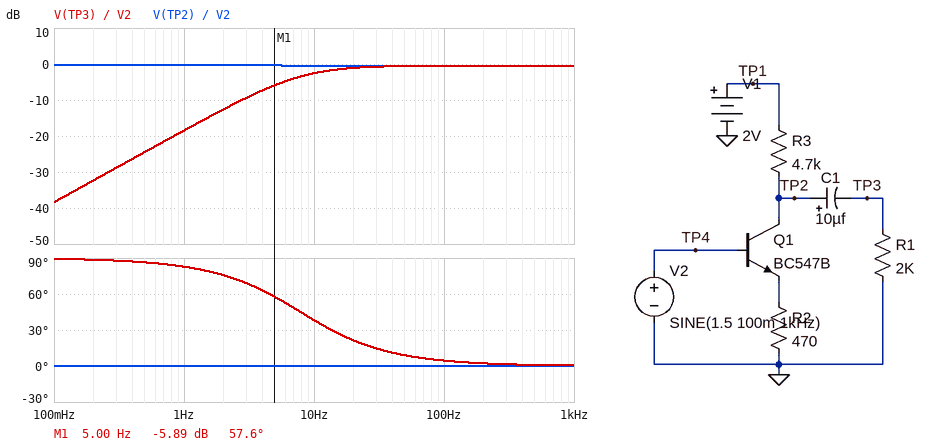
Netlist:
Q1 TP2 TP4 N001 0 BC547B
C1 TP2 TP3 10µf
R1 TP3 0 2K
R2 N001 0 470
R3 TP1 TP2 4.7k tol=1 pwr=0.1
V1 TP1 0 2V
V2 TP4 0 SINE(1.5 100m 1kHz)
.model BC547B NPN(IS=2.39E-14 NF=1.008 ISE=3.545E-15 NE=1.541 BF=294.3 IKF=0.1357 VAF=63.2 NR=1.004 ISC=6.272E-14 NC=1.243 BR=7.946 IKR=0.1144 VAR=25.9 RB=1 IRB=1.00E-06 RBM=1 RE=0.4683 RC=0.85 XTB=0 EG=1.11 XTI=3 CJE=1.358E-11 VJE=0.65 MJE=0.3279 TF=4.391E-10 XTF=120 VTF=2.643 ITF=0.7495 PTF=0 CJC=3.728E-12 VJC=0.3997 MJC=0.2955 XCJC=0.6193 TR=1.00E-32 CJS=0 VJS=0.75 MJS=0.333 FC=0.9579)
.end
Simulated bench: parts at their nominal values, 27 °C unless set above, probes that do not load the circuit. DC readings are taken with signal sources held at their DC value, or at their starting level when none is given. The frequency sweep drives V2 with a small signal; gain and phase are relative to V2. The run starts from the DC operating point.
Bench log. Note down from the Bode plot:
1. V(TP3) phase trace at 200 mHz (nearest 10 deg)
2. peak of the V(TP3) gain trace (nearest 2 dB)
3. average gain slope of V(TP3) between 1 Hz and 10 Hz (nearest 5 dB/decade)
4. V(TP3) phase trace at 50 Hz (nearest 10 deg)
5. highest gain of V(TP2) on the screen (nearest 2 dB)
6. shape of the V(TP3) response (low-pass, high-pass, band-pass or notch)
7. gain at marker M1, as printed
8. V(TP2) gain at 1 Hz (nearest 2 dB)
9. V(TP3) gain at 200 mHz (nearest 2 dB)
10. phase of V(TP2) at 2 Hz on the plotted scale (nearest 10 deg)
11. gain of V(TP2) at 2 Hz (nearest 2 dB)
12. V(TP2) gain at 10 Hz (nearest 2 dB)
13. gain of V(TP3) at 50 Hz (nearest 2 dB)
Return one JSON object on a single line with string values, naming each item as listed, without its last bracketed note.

{"V(TP3) phase trace at 200 mHz": "90 deg", "peak of the V(TP3) gain trace": "0 dB", "average gain slope of V(TP3) between 1 Hz and 10 Hz": "15 dB/decade", "V(TP3) phase trace at 50 Hz": "10 deg", "highest gain of V(TP2) on the screen": "0 dB", "shape of the V(TP3) response": "high-pass", "gain at marker M1, as printed": "-5.89 dB", "V(TP2) gain at 1 Hz": "0 dB", "V(TP3) gain at 200 mHz": "-32 dB", "phase of V(TP2) at 2 Hz on the plotted scale": "0 deg", "gain of V(TP2) at 2 Hz": "0 dB", "V(TP2) gain at 10 Hz": "0 dB", "gain of V(TP3) at 50 Hz": "0 dB"}
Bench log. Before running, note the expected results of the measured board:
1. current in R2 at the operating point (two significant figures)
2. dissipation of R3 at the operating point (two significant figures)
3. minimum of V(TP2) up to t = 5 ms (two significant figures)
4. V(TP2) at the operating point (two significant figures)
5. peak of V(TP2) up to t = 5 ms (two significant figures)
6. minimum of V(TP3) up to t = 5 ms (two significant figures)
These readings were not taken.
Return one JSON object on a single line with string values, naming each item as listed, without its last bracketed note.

{"current in R2 at the operating point": "1.7 mA", "dissipation of R3 at the operating point": "300 µW", "minimum of V(TP2) up to t = 5 ms": "710 mV", "V(TP2) at the operating point": "800 mV", "peak of V(TP2) up to t = 5 ms": "900 mV", "minimum of V(TP3) up to t = 5 ms": "-95 mV"}
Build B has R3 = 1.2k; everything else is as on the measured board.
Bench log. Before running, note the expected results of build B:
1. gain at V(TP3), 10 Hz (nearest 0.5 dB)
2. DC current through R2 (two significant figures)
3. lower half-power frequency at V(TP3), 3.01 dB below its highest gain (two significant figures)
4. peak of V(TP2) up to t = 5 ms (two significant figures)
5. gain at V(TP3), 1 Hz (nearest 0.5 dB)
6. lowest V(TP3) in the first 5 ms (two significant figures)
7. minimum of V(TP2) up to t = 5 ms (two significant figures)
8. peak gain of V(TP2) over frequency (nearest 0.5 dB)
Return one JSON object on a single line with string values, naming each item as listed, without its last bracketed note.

{"gain at V(TP3), 10 Hz": "-3.0 dB", "DC current through R2": "1.7 mA", "lower half-power frequency at V(TP3), 3.01 dB below its highest gain": "7.8 Hz", "peak of V(TP2) up to t = 5 ms": "910 mV", "gain at V(TP3), 1 Hz": "-19.0 dB", "lowest V(TP3) in the first 5 ms": "-86 mV", "minimum of V(TP2) up to t = 5 ms": "740 mV", "peak gain of V(TP2) over frequency": "-1.0 dB"}
